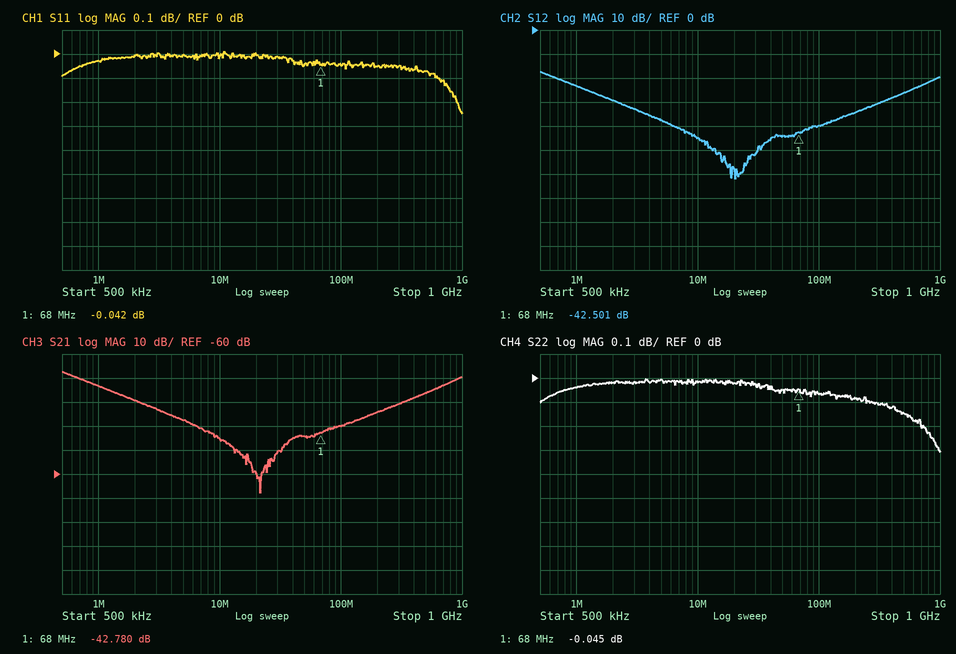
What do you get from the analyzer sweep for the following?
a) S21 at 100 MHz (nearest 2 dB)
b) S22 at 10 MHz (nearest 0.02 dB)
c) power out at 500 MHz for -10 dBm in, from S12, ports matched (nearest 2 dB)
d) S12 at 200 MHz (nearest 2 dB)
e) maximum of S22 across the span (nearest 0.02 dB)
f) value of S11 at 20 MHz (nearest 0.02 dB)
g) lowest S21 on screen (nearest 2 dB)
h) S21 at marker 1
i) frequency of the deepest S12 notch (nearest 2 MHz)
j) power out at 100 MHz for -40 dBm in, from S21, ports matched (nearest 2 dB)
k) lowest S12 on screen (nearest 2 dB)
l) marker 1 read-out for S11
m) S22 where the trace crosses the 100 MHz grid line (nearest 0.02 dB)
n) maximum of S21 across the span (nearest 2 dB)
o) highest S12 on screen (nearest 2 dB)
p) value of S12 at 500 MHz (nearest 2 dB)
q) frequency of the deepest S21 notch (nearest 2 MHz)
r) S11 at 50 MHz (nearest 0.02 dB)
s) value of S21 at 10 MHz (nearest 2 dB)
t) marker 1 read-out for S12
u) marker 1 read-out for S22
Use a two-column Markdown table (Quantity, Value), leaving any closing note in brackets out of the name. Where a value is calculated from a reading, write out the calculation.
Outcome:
| Quantity | Value |
|---|---|
| S21 at 100 MHz | -40 dB |
| S22 at 10 MHz | -0.02 dB |
| power out at 500 MHz for -10 dBm in, from S12, ports matched | -10 dBm + (-26 dB) = -36 dBm |
| S12 at 200 MHz | -34 dB |
| maximum of S22 across the span | 0.00 dB |
| value of S11 at 20 MHz | 0.00 dB |
| lowest S21 on screen | -68 dB |
| S21 at marker 1 | -42.780 dB |
| frequency of the deepest S12 notch | 20 MHz |
| power out at 100 MHz for -40 dBm in, from S21, ports matched | -40 dBm + (-40 dB) = -80 dBm |
| lowest S12 on screen | -62 dB |
| marker 1 read-out for S11 | -0.042 dB |
| S22 where the trace crosses the 100 MHz grid line | -0.06 dB |
| maximum of S21 across the span | -18 dB |
| highest S12 on screen | -18 dB |
| value of S12 at 500 MHz | -26 dB |
| frequency of the deepest S21 notch | 22 MHz |
| S11 at 50 MHz | -0.04 dB |
| value of S21 at 10 MHz | -46 dB |
| marker 1 read-out for S12 | -42.501 dB |
| marker 1 read-out for S22 | -0.045 dB |
